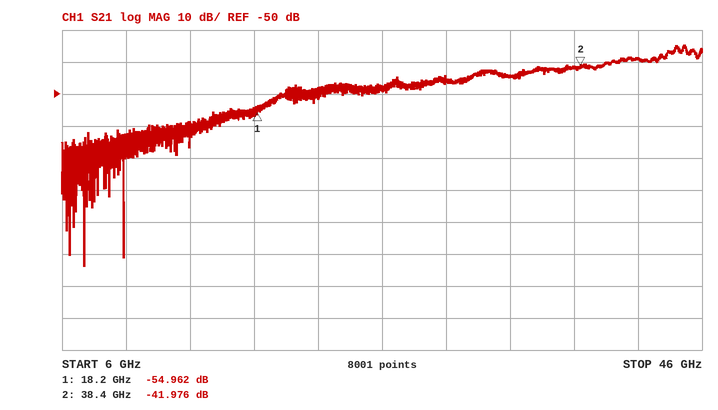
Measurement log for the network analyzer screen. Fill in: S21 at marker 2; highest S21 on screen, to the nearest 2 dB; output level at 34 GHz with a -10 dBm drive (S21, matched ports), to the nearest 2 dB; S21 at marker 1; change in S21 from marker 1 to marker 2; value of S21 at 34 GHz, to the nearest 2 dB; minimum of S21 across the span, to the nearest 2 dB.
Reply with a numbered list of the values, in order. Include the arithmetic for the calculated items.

1. -41.976 dB
2. -34 dB
3. -10 dBm + (-44 dB) = -54 dBm
4. -54.962 dB
5. -41.976 − (-54.962) = 12.986 dB
6. -44 dB
7. -104 dB
